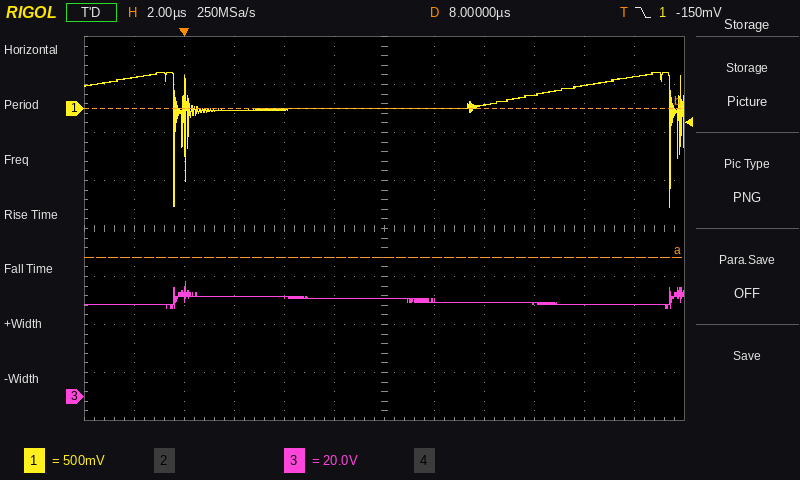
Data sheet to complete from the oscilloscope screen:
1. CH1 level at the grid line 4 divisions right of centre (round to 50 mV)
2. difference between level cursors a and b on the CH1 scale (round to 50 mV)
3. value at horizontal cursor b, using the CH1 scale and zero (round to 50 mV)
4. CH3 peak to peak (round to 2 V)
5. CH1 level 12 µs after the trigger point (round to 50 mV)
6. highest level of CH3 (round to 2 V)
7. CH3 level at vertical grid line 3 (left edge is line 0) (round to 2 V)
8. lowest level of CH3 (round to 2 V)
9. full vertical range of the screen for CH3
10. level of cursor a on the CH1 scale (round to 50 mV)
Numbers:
250 mV
1.55 V
0 mV
12 V
50 mV
48 V
42 V
36 V
160 V
-1.55 V
